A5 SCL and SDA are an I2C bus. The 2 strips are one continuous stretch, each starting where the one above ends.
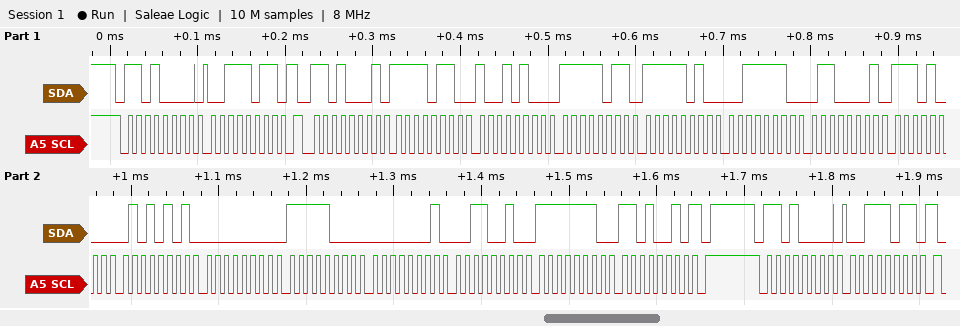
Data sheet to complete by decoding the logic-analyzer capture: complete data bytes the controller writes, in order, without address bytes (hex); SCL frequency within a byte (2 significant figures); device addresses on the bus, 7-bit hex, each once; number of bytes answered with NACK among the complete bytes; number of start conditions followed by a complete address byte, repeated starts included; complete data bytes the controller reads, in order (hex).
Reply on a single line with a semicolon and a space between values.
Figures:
3B 3B; 100 kHz; 0x68; 1; 3; F6 94 FB FA 3E 61 E8 55 00 F8 01 32 FE D2
